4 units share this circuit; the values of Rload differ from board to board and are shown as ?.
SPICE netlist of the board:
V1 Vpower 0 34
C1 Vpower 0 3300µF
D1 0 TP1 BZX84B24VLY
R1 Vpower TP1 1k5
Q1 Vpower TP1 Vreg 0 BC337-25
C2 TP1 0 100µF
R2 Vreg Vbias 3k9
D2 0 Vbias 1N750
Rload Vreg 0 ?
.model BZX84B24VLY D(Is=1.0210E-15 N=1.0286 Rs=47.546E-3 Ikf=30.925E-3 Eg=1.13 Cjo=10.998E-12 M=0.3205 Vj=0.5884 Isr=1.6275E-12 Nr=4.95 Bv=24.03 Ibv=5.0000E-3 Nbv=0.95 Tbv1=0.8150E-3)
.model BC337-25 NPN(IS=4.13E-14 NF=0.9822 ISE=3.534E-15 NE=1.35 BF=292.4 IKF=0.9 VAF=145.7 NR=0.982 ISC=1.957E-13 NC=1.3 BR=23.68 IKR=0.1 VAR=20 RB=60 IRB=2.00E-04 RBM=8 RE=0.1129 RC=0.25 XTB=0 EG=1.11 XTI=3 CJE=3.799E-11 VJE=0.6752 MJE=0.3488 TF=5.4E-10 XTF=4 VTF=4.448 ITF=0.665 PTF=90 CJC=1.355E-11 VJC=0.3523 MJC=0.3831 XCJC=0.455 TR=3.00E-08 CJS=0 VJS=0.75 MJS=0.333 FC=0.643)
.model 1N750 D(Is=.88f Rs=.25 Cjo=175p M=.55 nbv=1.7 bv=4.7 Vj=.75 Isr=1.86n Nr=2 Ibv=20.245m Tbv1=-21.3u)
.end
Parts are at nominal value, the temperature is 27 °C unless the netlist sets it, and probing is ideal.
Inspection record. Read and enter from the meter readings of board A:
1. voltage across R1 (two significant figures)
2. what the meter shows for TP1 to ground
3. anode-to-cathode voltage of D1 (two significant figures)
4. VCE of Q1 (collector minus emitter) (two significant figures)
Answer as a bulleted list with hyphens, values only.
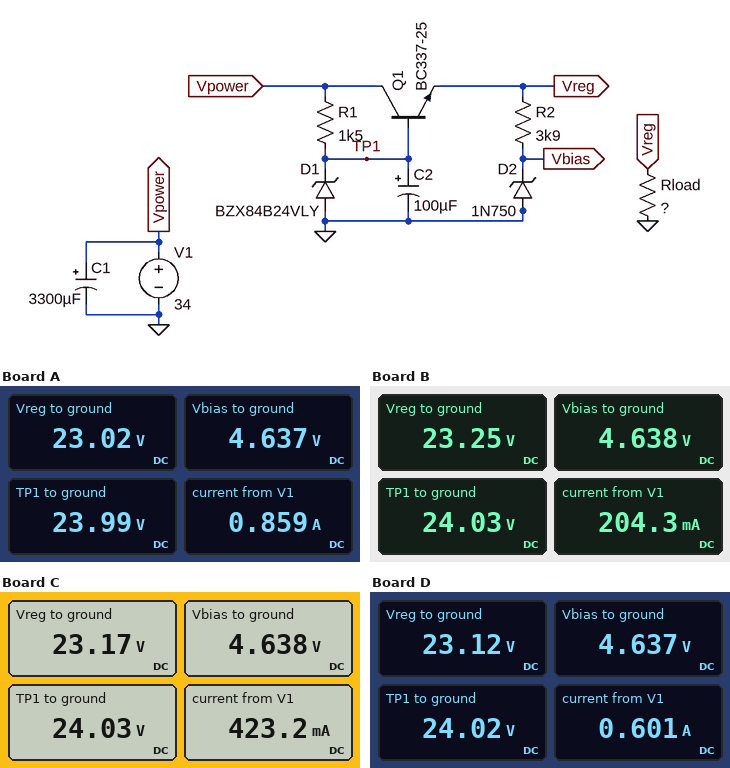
- 10 V
- 23.99 V
- -24 V
- 11 V
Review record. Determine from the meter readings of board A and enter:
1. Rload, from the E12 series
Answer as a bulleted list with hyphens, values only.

- 27 Ω
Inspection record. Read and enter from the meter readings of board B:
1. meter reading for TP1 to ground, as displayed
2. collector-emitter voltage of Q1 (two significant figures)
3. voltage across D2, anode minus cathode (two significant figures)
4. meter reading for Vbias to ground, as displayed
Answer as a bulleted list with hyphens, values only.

- 24.03 V
- 11 V
- -4.6 V
- 4.638 V
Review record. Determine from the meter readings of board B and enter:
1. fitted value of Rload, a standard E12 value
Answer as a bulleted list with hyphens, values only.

- 120 Ω
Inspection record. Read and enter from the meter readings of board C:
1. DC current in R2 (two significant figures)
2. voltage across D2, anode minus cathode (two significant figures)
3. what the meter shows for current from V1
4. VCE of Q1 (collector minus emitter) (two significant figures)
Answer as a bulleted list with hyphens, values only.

- 4.8 mA
- -4.6 V
- 423.2 mA
- 11 V
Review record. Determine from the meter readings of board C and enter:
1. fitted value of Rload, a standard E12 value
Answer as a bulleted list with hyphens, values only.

- 56 Ω
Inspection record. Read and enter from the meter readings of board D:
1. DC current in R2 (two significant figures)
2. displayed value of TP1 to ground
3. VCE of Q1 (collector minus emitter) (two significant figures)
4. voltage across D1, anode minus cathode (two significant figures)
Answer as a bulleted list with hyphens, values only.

- 4.7 mA
- 24.02 V
- 11 V
- -24 V
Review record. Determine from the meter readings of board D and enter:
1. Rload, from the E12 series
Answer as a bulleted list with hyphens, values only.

- 39 Ω
